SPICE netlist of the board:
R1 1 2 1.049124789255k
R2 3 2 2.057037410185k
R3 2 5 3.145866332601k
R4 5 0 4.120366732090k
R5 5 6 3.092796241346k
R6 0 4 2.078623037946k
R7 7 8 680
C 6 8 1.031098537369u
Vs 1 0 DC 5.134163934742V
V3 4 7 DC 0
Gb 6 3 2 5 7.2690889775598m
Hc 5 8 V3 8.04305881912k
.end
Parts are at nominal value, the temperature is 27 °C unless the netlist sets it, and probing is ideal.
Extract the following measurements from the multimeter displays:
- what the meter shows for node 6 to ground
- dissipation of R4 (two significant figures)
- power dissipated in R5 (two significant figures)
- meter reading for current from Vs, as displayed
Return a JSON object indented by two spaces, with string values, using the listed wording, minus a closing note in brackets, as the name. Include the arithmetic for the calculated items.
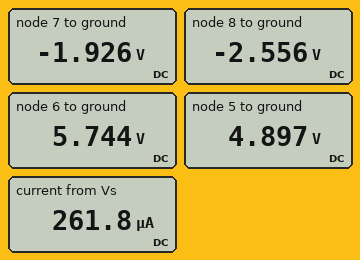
{
  "what the meter shows for node 6 to ground": "5.744 V",
  "dissipation of R4": "(4.897 V)^2 / 4.12 kΩ = 5.8 mW",
  "power dissipated in R5": "(5.744 V - 4.897 V)^2 / 3.093 kΩ = 230 µW",
  "meter reading for current from Vs, as displayed": "261.8 µA"
}
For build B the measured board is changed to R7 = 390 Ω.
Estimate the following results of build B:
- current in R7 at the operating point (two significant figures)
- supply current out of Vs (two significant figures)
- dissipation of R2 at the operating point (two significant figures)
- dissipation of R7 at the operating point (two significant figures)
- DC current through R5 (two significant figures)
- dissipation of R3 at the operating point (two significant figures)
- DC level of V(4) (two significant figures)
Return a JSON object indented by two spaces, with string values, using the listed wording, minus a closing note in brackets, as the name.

{
  "current in R7 at the operating point": "870 µA",
  "supply current out of Vs": "310 µA",
  "dissipation of R2 at the operating point": "210 µW",
  "dissipation of R7 at the operating point": "300 µW",
  "DC current through R5": "320 µA",
  "dissipation of R3 at the operating point": "620 nW",
  "DC level of V(4)": "-1.8 V"
}
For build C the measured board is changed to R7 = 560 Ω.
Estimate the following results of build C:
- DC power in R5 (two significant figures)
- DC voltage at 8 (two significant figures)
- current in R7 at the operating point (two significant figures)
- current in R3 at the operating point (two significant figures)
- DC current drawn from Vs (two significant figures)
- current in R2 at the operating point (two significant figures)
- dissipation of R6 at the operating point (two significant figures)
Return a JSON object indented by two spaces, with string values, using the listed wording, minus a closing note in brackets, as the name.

{
  "DC power in R5": "270 µW",
  "DC voltage at 8": "-2.4 V",
  "current in R7 at the operating point": "900 µA",
  "current in R3 at the operating point": "13 µA",
  "DC current drawn from Vs": "280 µA",
  "current in R2 at the operating point": "290 µA",
  "dissipation of R6 at the operating point": "1.7 mW"
}
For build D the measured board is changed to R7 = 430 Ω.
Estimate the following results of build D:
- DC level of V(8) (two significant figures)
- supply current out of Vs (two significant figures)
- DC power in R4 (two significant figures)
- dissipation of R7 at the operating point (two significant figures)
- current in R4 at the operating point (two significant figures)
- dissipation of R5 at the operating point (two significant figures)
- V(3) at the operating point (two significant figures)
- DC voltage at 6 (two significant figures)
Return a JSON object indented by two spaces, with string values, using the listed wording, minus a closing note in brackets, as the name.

{
  "DC level of V(8)": "-2.2 V",
  "supply current out of Vs": "300 µA",
  "DC power in R4": "5.7 mW",
  "dissipation of R7 at the operating point": "330 µW",
  "current in R4 at the operating point": "1.2 mA",
  "dissipation of R5 at the operating point": "310 µW",
  "V(3) at the operating point": "4.2 V",
  "DC voltage at 6": "5.8 V"
}
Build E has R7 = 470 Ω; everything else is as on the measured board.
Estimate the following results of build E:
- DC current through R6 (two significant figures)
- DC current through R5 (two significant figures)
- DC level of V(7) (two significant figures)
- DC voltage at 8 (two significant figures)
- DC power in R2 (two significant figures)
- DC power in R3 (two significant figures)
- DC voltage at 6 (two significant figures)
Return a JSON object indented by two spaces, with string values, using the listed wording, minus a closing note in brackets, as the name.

{
  "DC current through R6": "890 µA",
  "DC current through R5": "310 µA",
  "DC level of V(7)": "-1.8 V",
  "DC voltage at 8": "-2.3 V",
  "DC power in R2": "200 µW",
  "DC power in R3": "570 nW",
  "DC voltage at 6": "5.8 V"
}
